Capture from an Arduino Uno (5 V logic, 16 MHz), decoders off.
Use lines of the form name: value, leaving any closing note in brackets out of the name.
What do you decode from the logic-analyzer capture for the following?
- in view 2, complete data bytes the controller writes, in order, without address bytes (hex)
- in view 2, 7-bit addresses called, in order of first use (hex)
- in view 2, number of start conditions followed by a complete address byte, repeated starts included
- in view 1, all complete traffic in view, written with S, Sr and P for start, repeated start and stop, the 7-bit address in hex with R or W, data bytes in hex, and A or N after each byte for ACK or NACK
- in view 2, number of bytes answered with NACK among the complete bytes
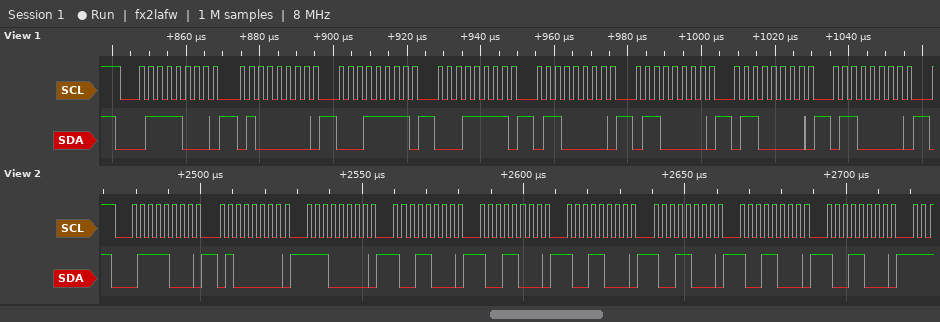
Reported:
in view 2, complete data bytes the controller writes, in order, without address bytes: 40 E0 98 98 98 98 98 98
in view 2, 7-bit addresses called, in order of first use: 0x3C
in view 2, number of start conditions followed by a complete address byte, repeated starts included: 1
in view 1, all complete traffic in view, written with S, Sr and P for start, repeated start and stop, the 7-bit address in hex with R or W, data bytes in hex, and A or N after each byte for ACK or NACK: S 3CW A 40 A 1F A 1F A 60 A 60 A 60 A 60 A
in view 2, number of bytes answered with NACK among the complete bytes: 0
